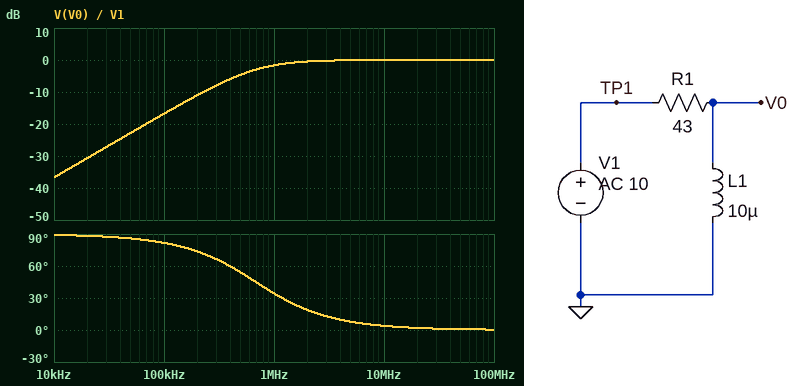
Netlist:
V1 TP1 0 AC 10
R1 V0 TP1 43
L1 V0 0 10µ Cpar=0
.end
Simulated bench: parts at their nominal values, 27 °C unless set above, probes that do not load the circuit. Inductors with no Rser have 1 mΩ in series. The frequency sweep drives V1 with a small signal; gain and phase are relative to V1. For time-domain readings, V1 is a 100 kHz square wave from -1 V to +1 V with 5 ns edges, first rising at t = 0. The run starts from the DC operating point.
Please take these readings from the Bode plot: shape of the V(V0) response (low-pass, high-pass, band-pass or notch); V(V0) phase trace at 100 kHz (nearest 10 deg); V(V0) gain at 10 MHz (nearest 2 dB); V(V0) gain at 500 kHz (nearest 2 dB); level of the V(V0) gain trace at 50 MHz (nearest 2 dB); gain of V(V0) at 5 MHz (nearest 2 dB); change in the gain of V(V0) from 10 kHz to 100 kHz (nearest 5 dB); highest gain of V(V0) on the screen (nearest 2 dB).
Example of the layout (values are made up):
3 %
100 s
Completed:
high-pass
80 deg
0 dB
-4 dB
0 dB
0 dB
20 dB
0 dB
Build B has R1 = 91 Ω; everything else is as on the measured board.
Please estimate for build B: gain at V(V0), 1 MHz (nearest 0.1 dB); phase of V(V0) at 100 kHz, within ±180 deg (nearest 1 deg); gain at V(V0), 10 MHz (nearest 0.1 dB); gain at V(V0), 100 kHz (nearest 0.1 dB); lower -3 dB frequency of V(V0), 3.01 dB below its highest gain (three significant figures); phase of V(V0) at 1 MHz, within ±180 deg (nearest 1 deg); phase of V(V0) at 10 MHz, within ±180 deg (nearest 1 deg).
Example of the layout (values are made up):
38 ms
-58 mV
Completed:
-4.9 dB
86 deg
-0.1 dB
-23.2 dB
1.45 MHz
55 deg
8 deg
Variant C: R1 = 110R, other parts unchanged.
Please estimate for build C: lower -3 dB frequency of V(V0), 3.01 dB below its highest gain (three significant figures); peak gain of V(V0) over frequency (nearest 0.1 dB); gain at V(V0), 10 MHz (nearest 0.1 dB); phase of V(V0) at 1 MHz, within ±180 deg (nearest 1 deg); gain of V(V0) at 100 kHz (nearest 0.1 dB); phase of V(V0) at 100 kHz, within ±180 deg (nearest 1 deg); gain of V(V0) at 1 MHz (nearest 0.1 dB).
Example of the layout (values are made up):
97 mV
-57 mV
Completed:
1.75 MHz
0 dB
-0.1 dB
60 deg
-24.9 dB
87 deg
-6.1 dB
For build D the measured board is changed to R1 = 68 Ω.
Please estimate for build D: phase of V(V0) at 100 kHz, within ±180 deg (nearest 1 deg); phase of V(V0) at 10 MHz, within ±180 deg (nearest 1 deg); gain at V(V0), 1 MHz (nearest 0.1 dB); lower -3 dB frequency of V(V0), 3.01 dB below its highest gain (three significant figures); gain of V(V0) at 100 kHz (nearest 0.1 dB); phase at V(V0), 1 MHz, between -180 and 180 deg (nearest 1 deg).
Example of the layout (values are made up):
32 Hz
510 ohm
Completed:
85 deg
6 deg
-3.4 dB
1.08 MHz
-20.7 dB
47 deg
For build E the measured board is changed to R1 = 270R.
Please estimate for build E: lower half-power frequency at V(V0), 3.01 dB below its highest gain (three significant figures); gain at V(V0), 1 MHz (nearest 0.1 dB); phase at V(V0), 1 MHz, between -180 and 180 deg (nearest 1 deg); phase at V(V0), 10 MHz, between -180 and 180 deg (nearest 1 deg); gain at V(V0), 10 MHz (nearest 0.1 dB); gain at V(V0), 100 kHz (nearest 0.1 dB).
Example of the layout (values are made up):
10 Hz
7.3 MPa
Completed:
4.30 MHz
-12.9 dB
77 deg
23 deg
-0.7 dB
-32.7 dB
